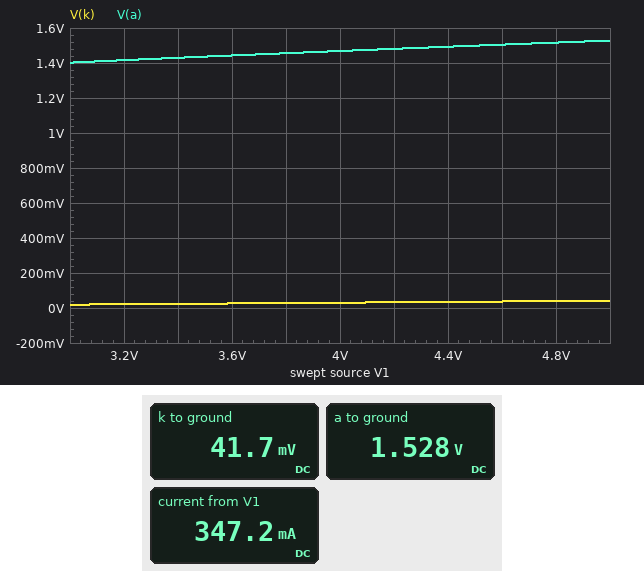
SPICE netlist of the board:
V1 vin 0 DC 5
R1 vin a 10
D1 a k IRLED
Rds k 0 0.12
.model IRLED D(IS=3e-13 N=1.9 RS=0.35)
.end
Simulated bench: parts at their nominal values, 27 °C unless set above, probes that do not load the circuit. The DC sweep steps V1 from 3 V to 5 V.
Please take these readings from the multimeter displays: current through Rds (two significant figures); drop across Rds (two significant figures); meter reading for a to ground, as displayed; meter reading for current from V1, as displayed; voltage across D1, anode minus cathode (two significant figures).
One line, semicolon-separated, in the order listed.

350 mA; 42 mV; 1.528 V; 347.2 mA; 1.5 V
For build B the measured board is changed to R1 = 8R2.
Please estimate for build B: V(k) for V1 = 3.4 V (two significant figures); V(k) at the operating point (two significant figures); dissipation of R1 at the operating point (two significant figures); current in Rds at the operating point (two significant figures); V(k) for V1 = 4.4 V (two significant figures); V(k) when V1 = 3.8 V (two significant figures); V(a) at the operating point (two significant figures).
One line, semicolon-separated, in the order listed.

28 mV; 50 mV; 1.4 W; 420 mA; 42 mV; 34 mV; 1.6 V
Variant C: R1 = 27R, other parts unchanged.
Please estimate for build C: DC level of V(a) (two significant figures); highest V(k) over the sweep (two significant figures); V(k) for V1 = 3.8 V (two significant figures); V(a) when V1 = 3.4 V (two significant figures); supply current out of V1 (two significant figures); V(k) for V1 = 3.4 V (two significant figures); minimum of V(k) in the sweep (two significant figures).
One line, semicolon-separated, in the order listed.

1.4 V; 16 mV; 11 mV; 1.3 V; 130 mA; 9.2 mV; 7.5 mV
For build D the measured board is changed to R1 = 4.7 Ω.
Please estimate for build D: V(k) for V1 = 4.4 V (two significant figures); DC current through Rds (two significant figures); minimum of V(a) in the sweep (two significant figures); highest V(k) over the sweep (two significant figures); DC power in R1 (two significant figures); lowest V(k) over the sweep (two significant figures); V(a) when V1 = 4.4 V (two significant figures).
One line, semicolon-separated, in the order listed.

70 mV; 700 mA; 1.5 V; 84 mV; 2.3 W; 38 mV; 1.7 V
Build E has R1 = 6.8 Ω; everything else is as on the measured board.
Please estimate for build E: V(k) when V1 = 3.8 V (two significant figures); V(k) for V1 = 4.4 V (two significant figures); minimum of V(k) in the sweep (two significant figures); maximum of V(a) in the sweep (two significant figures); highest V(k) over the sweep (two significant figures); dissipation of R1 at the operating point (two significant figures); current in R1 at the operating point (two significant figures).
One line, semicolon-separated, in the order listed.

40 mV; 50 mV; 27 mV; 1.6 V; 60 mV; 1.7 W; 500 mA
